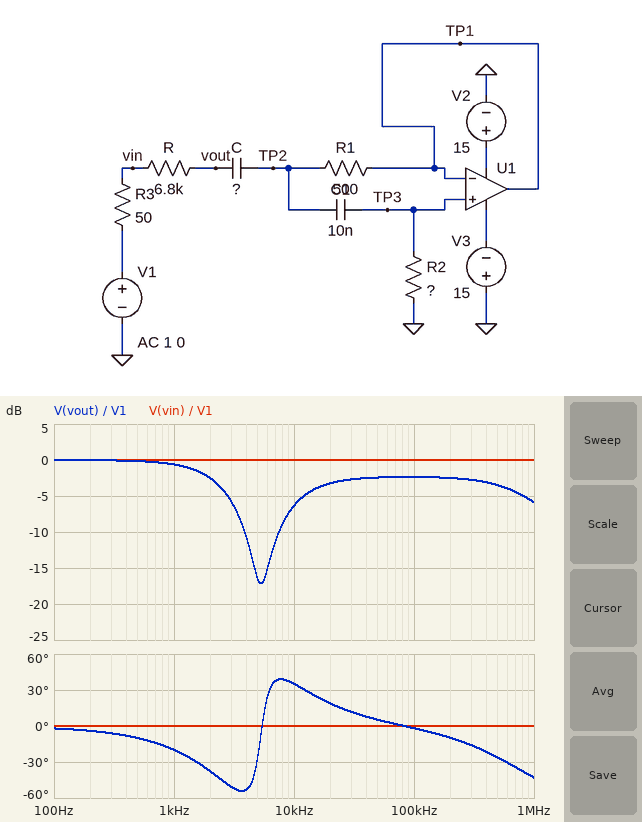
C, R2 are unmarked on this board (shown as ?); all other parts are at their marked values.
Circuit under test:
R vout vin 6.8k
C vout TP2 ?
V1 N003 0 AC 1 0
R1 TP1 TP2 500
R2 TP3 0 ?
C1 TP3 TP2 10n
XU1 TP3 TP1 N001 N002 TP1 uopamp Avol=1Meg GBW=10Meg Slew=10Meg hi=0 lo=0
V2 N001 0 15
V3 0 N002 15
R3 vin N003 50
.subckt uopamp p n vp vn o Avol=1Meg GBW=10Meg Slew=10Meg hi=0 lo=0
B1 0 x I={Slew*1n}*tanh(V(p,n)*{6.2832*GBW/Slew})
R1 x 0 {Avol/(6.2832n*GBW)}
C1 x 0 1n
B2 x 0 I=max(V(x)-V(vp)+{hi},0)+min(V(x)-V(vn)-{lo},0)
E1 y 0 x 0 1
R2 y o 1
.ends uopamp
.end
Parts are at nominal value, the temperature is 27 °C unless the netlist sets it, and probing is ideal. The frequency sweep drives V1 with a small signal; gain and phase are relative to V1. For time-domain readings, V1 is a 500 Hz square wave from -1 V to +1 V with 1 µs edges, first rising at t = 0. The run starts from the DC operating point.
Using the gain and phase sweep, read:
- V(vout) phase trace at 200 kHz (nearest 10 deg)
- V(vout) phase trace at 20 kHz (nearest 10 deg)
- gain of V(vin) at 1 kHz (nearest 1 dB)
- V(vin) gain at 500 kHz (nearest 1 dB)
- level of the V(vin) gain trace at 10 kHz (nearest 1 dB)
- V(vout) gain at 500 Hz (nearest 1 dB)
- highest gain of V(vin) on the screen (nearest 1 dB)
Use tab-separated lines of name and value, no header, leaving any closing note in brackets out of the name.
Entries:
V(vout) phase trace at 200 kHz	-10 deg
V(vout) phase trace at 20 kHz	20 deg
gain of V(vin) at 1 kHz	0 dB
V(vin) gain at 500 kHz	0 dB
level of the V(vin) gain trace at 10 kHz	0 dB
V(vout) gain at 500 Hz	0 dB
highest gain of V(vin) on the screen	0 dB
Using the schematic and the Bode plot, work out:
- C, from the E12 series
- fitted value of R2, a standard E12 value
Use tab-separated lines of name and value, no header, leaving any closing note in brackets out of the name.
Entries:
C, from the E12 series	8.2 nF
fitted value of R2, a standard E12 value	22 kΩ
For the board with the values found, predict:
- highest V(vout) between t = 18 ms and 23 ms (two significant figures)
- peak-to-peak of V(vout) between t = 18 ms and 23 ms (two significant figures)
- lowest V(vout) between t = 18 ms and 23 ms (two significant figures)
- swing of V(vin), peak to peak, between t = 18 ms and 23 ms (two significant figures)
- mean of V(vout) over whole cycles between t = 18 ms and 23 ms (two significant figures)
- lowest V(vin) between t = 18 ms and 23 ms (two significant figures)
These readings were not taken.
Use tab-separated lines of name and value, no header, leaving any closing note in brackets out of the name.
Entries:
highest V(vout) between t = 18 ms and 23 ms	1.0 V
peak-to-peak of V(vout) between t = 18 ms and 23 ms	2.0 V
lowest V(vout) between t = 18 ms and 23 ms	-1.0 V
swing of V(vin), peak to peak, between t = 18 ms and 23 ms	2.0 V
mean of V(vout) over whole cycles between t = 18 ms and 23 ms	170 mV
lowest V(vin) between t = 18 ms and 23 ms	-1.0 V
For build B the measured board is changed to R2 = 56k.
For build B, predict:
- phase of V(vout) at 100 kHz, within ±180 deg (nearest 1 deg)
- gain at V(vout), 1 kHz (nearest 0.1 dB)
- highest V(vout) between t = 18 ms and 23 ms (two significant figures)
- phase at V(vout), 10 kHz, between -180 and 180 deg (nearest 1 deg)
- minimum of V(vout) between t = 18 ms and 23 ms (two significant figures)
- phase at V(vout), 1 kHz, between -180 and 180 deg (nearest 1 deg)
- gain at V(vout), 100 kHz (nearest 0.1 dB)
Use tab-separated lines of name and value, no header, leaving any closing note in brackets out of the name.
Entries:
phase of V(vout) at 100 kHz, within ±180 deg	-5 deg
gain at V(vout), 1 kHz	-0.7 dB
highest V(vout) between t = 18 ms and 23 ms	1.1 V
phase at V(vout), 10 kHz, between -180 and 180 deg	19 deg
minimum of V(vout) between t = 18 ms and 23 ms	-1.1 V
phase at V(vout), 1 kHz, between -180 and 180 deg	-21 deg
gain at V(vout), 100 kHz	-1.0 dB
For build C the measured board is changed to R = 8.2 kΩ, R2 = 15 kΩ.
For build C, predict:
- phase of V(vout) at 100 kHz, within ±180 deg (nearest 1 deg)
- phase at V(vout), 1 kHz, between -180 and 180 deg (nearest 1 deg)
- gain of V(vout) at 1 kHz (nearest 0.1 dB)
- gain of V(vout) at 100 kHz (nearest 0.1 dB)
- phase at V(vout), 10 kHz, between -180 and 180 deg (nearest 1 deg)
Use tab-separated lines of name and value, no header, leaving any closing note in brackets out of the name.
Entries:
phase of V(vout) at 100 kHz, within ±180 deg	0 deg
phase at V(vout), 1 kHz, between -180 and 180 deg	-23 deg
gain of V(vout) at 1 kHz	-0.8 dB
gain of V(vout) at 100 kHz	-3.8 dB
phase at V(vout), 10 kHz, between -180 and 180 deg	38 deg
